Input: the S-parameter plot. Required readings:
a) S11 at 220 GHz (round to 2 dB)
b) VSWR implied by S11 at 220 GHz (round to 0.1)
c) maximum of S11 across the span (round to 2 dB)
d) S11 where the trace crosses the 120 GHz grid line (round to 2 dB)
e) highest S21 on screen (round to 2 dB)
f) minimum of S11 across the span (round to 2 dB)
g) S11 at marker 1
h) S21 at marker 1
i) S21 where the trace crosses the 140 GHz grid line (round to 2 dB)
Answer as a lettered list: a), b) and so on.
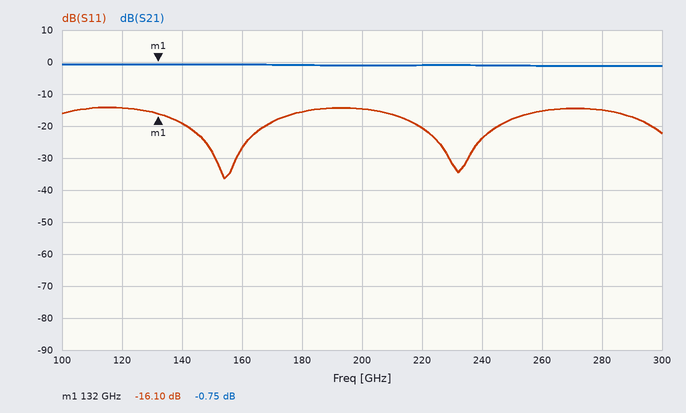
a) -20 dB
b) 1.2
c) -14 dB
d) -14 dB
e) 0 dB
f) -36 dB
g) -16.10 dB
h) -0.75 dB
i) 0 dB
